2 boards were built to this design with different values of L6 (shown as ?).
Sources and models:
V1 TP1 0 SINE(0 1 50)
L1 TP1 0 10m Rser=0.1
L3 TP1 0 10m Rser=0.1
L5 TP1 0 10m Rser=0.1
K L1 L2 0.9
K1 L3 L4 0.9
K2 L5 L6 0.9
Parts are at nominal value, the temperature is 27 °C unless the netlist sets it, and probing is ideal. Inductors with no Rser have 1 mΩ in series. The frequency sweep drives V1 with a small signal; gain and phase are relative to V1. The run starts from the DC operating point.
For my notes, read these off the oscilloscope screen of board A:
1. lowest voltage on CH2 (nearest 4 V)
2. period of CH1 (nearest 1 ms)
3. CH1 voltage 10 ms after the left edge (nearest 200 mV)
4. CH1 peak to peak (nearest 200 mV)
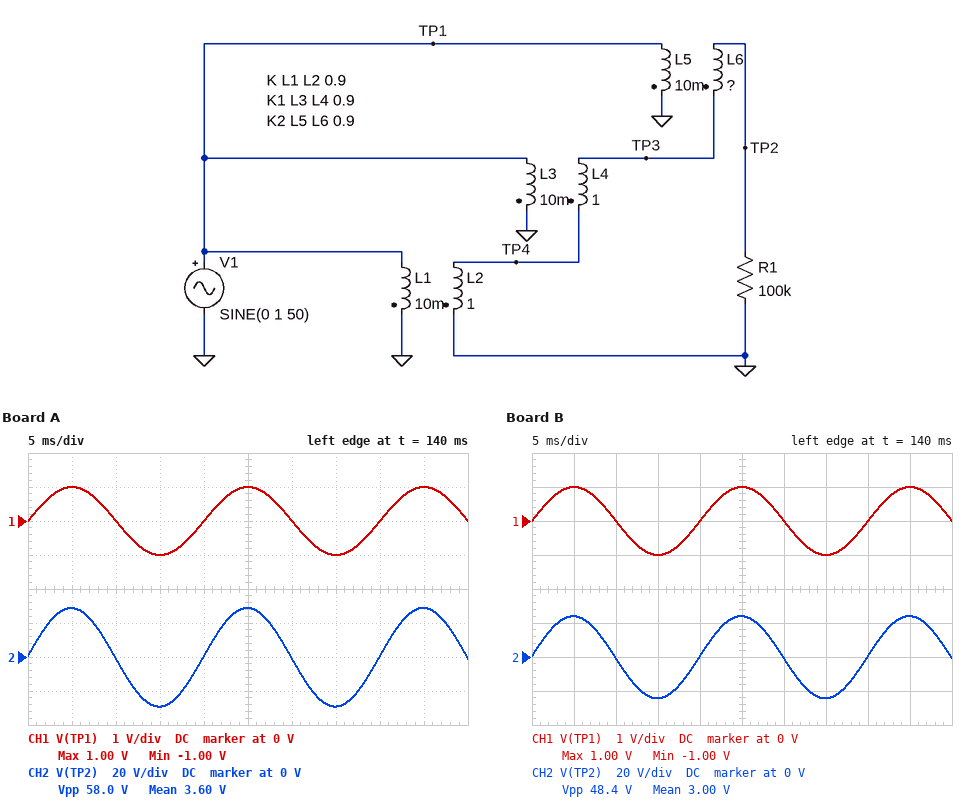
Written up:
-28 V
20 ms
0 V
2.0 V
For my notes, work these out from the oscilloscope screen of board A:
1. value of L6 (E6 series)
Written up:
1.5 H
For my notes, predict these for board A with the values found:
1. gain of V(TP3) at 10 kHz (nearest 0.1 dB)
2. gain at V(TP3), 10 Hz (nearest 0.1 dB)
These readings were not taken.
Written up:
24.4 dB
25.0 dB
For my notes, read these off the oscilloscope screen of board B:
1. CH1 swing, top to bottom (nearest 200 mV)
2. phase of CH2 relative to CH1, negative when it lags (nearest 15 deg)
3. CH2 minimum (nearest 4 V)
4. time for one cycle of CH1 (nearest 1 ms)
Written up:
2.0 V
0 deg
-24 V
20 ms
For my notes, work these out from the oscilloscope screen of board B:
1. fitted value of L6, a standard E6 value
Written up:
470 mH
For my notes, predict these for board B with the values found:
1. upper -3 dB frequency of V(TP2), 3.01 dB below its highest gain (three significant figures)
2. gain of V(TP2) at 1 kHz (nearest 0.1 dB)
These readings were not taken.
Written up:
33.9 kHz
27.7 dB
